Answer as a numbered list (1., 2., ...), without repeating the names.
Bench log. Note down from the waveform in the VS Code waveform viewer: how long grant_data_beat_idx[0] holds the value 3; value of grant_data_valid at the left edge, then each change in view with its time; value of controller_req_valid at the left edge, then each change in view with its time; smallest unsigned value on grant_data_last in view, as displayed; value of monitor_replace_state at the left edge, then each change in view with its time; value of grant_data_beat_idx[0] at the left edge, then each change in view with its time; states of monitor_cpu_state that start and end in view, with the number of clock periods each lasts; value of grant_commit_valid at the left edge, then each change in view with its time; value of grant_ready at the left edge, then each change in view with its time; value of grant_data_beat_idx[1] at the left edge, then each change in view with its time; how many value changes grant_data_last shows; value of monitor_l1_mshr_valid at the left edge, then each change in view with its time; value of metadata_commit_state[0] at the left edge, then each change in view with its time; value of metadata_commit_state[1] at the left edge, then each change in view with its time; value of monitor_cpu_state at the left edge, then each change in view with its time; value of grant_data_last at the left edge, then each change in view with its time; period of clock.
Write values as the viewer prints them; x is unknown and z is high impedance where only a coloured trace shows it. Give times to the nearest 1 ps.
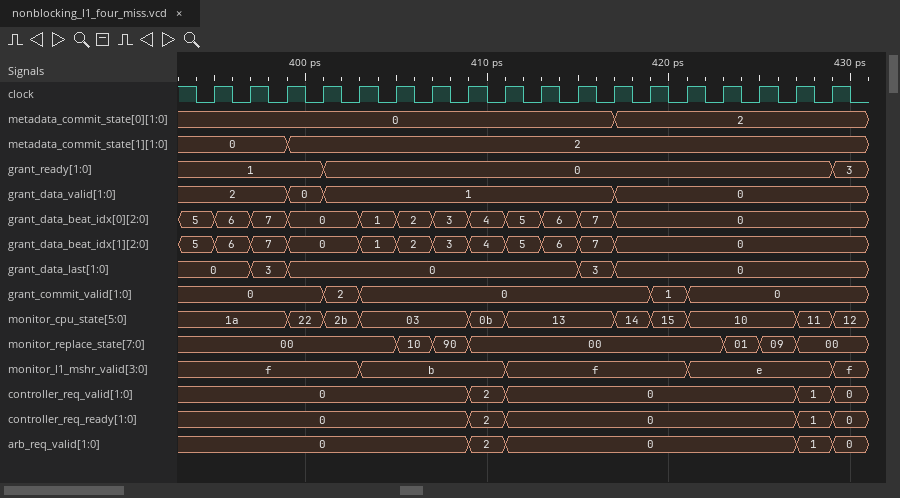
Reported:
1. 2 ps
2. 2, 0 at 399 ps, 1 at 401 ps, 0 at 417 ps
3. 0, 2 at 409 ps, 0 at 411 ps, 1 at 427 ps, 0 at 429 ps
4. 0
5. 00, 10 at 405 ps, 90 at 407 ps, 00 at 409 ps, 01 at 423 ps, 09 at 425 ps, 00 at 427 ps
6. 5, 6 at 395 ps, 7 at 397 ps, 0 at 399 ps, 1 at 403 ps, 2 at 405 ps, 3 at 407 ps, 4 at 409 ps, 5 at 411 ps, 6 at 413 ps, 7 at 415 ps, 0 at 417 ps
7. 22: 1, 2b: 1, 03: 3, 0b: 1, 13: 3, 14: 1, 15: 1, 10: 3, 11: 1
8. 0, 2 at 401 ps, 0 at 403 ps, 1 at 419 ps, 0 at 421 ps
9. 1, 0 at 401 ps, 3 at 429 ps
10. 5, 6 at 395 ps, 7 at 397 ps, 0 at 399 ps, 1 at 403 ps, 2 at 405 ps, 3 at 407 ps, 4 at 409 ps, 5 at 411 ps, 6 at 413 ps, 7 at 415 ps, 0 at 417 ps
11. 4
12. f, b at 403 ps, f at 411 ps, e at 421 ps, f at 429 ps
13. 0, 2 at 417 ps
14. 0, 2 at 399 ps
15. 1a, 22 at 399 ps, 2b at 401 ps, 03 at 403 ps, 0b at 409 ps, 13 at 411 ps, 14 at 417 ps, 15 at 419 ps, 10 at 421 ps, 11 at 427 ps, 12 at 429 ps
16. 0, 3 at 397 ps, 0 at 399 ps, 3 at 415 ps, 0 at 417 ps
17. 2 ps
